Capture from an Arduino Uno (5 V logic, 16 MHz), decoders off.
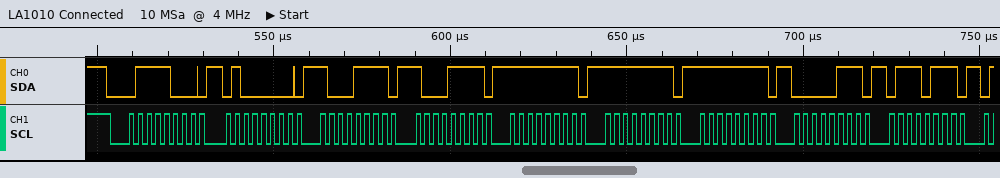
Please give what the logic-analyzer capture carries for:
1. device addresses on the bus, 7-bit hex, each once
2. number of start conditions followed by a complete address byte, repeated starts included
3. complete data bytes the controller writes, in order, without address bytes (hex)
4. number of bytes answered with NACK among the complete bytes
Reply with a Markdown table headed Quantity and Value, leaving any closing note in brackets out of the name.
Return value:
| Quantity | Value |
|---|---|
| device addresses on the bus, 7-bit hex, each once | 0x3C |
| number of start conditions followed by a complete address byte, repeated starts included | 1 |
| complete data bytes the controller writes, in order, without address bytes | 40 8F 8F FF FF FF 07 77 |
| number of bytes answered with NACK among the complete bytes | 0 |
